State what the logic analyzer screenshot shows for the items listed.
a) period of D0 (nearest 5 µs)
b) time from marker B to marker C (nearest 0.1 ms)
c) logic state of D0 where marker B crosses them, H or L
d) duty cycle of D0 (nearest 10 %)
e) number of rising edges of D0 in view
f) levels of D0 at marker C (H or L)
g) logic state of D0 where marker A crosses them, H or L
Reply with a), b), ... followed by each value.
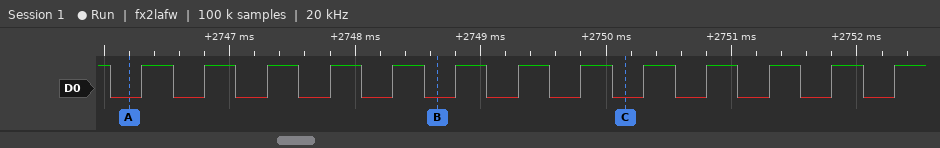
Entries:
a) 500 µs
b) 1.5 ms
c) D0=L
d) 50 %
e) 13
f) D0=L
g) D0=L
